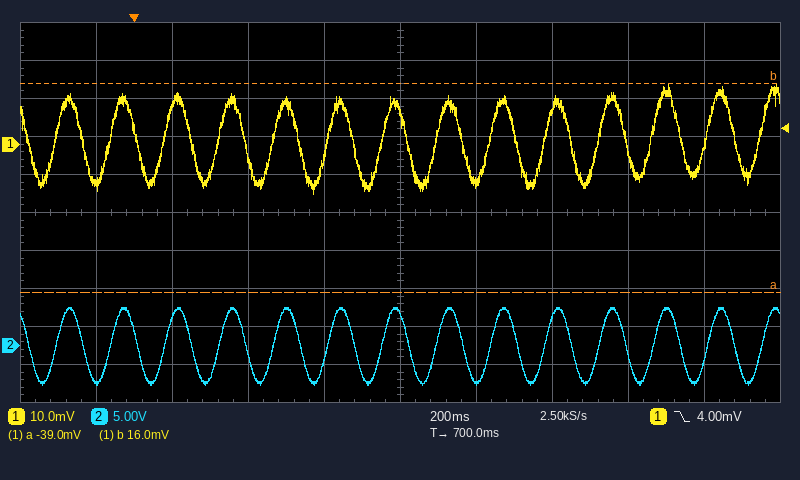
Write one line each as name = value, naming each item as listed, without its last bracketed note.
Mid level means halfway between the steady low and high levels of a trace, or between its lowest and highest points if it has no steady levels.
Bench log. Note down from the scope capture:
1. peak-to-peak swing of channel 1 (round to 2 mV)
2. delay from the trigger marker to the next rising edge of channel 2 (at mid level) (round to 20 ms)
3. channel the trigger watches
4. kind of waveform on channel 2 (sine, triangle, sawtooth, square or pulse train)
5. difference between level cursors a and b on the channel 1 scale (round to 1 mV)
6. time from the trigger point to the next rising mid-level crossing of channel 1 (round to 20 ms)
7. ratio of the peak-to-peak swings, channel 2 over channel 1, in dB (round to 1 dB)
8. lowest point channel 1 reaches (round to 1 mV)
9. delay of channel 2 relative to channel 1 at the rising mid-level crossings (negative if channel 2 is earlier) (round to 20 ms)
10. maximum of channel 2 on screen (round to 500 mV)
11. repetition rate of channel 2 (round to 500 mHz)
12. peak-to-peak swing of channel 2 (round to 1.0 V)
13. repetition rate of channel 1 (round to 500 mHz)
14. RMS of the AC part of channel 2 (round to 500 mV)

peak-to-peak swing of channel 1 = 28 mV
delay from the trigger marker to the next rising edge of channel 2 (at mid level) = 80 ms
channel the trigger watches = channel 1
kind of waveform on channel 2 = sine
difference between level cursors a and b on the channel 1 scale = 55 mV
time from the trigger point to the next rising mid-level crossing of channel 1 = 80 ms
ratio of the peak-to-peak swings, channel 2 over channel 1, in dB = 51 dB
lowest point channel 1 reaches = -13 mV
delay of channel 2 relative to channel 1 at the rising mid-level crossings (negative if channel 2 is earlier) = 0 ms
maximum of channel 2 on screen = 5.0 V
repetition rate of channel 2 = 7.0 Hz
peak-to-peak swing of channel 2 = 10.0 V
repetition rate of channel 1 = 7.0 Hz
RMS of the AC part of channel 2 = 3.5 V
